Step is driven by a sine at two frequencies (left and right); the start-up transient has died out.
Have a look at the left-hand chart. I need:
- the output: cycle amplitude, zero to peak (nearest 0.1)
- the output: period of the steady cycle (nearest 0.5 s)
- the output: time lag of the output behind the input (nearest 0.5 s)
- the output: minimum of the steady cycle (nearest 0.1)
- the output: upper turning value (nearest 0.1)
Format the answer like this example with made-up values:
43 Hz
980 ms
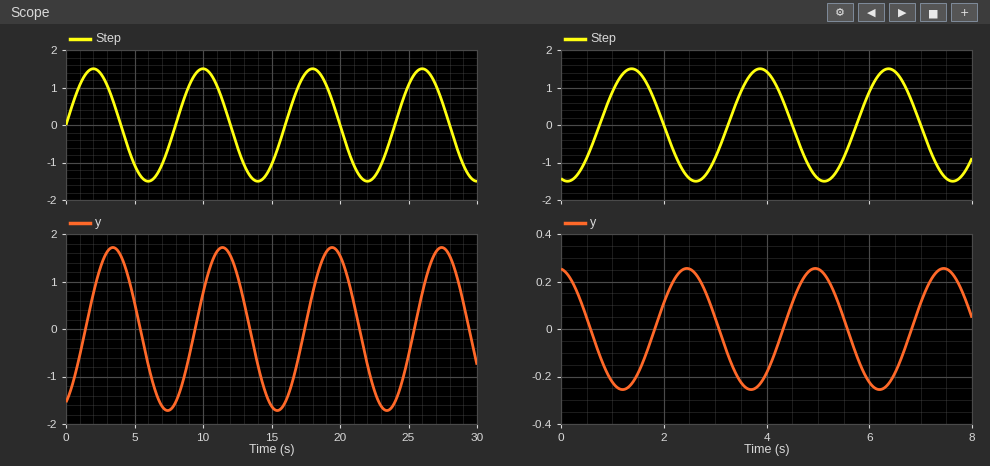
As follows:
1.7
8.0 s
1.5 s
-1.7
1.7
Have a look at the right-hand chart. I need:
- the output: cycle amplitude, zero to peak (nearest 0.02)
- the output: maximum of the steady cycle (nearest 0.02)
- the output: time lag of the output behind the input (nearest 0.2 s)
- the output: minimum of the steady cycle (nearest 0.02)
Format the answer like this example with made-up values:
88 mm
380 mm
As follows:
0.26
0.26
1.0 s
-0.26
